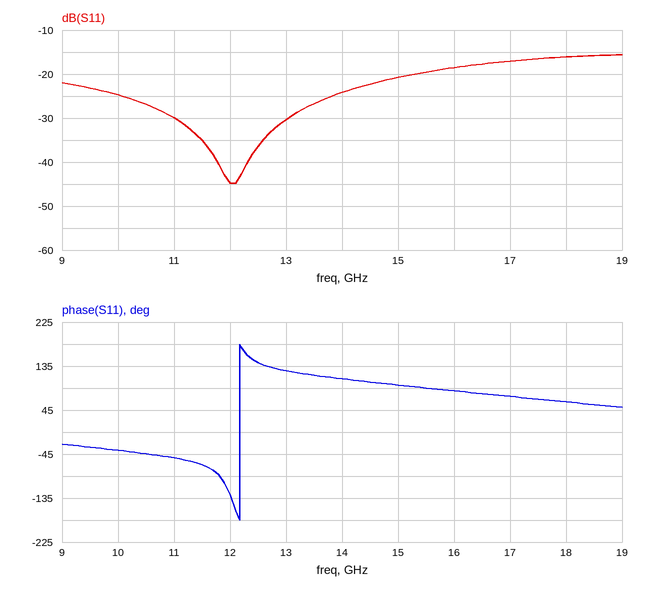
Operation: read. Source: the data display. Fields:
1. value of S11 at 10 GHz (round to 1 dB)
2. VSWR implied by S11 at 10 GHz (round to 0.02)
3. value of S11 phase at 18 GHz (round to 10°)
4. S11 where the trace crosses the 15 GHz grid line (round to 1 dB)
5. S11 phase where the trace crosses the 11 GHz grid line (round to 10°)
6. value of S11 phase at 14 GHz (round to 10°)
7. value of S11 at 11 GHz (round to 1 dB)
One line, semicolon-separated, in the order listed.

-25 dB; 1.12; 60°; -21 dB; -50°; 110°; -30 dB
